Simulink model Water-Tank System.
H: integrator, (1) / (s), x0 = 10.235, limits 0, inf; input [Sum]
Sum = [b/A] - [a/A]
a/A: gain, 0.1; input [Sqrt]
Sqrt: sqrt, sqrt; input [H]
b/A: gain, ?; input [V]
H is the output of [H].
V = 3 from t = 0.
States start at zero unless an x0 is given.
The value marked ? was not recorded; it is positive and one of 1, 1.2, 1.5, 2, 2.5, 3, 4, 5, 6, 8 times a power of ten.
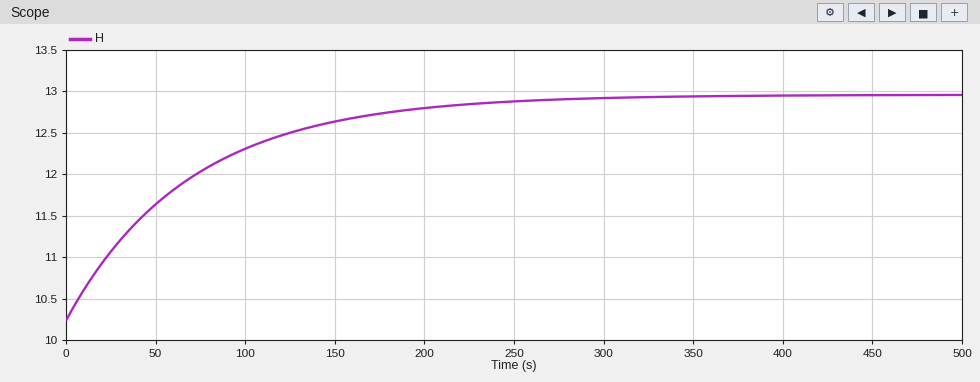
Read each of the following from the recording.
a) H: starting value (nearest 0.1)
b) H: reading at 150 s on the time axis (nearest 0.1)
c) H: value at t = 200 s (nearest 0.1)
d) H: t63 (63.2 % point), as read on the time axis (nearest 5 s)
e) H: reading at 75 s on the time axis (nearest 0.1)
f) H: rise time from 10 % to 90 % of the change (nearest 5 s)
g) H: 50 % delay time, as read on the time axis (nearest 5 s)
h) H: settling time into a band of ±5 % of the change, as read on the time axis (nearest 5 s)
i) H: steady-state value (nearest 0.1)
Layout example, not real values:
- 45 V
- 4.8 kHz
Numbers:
- 10.2
- 12.6
- 12.8
- 70 s
- 12.0
- 155 s
- 50 s
- 210 s
- 13.0
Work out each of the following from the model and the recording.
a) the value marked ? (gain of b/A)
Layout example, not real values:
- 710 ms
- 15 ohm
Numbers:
- 0.12
